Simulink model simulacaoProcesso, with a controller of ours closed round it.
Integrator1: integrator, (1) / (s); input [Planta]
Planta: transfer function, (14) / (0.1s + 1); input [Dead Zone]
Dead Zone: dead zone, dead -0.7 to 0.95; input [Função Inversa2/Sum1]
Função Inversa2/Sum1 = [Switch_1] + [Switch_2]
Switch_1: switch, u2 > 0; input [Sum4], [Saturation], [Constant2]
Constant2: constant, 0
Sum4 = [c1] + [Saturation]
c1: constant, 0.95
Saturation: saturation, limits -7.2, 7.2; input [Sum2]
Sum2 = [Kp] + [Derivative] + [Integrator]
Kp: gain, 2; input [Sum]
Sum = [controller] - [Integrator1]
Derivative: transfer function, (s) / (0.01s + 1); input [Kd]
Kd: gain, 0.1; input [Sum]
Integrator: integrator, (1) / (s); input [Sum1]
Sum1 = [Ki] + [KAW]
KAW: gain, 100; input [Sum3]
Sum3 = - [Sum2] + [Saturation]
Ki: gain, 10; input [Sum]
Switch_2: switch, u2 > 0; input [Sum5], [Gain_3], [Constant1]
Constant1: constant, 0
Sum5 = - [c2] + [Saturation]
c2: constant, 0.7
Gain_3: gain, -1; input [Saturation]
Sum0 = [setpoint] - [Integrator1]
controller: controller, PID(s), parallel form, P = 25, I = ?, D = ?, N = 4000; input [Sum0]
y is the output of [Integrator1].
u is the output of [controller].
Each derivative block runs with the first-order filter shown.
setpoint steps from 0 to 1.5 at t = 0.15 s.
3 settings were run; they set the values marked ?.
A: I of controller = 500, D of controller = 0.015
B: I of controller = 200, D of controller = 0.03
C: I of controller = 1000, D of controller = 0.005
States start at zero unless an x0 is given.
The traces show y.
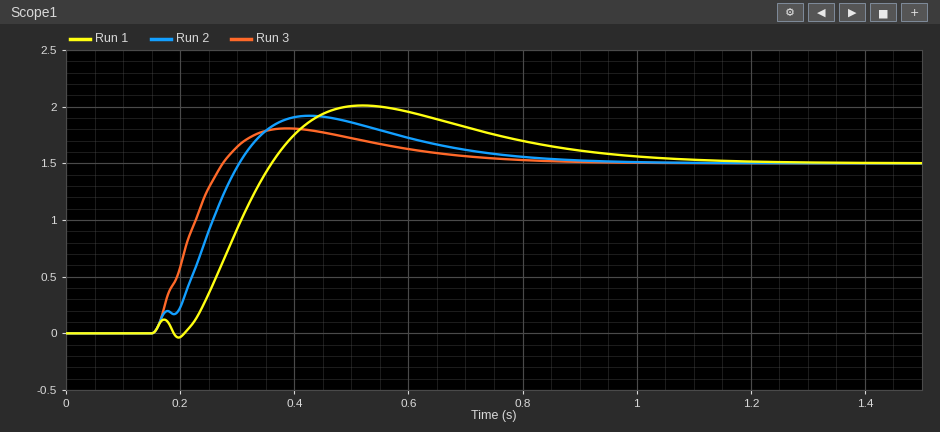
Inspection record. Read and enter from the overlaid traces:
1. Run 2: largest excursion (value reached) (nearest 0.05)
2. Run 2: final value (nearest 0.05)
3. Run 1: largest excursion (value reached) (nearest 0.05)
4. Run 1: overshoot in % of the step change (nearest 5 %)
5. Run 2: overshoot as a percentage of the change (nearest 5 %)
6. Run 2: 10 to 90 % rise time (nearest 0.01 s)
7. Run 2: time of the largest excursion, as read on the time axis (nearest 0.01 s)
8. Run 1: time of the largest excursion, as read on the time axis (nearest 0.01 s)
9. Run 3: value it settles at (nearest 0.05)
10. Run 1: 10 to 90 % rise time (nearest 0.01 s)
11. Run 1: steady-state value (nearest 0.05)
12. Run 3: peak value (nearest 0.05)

1.90
1.50
2.00
35 %
30 %
0.12 s
0.43 s
0.52 s
1.50
0.11 s
1.50
1.80
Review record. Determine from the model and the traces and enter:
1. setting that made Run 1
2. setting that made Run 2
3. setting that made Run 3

B
A
C
